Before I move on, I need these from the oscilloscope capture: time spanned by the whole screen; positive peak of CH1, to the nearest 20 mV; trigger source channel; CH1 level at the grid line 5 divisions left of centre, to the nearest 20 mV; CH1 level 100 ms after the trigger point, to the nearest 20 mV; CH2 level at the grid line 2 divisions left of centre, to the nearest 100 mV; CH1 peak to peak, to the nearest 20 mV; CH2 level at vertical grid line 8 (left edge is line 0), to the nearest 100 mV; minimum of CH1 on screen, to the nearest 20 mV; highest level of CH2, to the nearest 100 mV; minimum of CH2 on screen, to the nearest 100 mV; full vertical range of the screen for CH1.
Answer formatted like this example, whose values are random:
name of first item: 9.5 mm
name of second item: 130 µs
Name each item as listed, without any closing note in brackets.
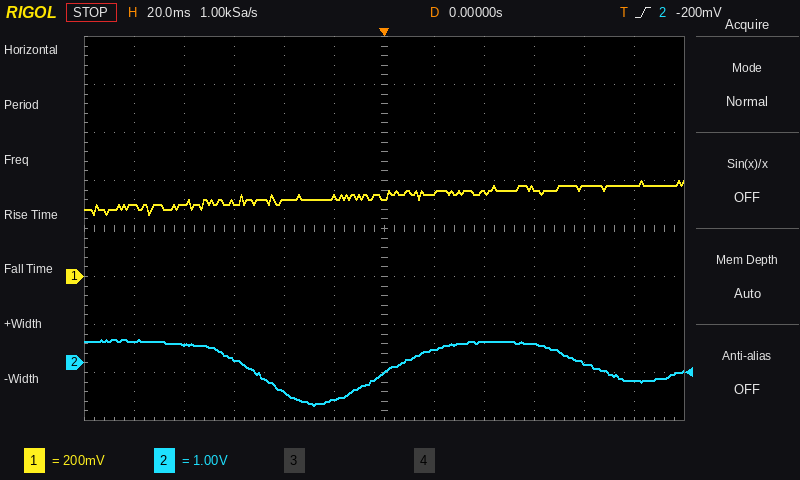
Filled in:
time spanned by the whole screen: 240 ms
positive peak of CH1, to the nearest 20 mV: 400 mV
trigger source channel: CH2
CH1 level at the grid line 5 divisions left of centre, to the nearest 20 mV: 300 mV
CH1 level 100 ms after the trigger point, to the nearest 20 mV: 380 mV
CH2 level at the grid line 2 divisions left of centre, to the nearest 100 mV: -600 mV
CH1 peak to peak, to the nearest 20 mV: 140 mV
CH2 level at vertical grid line 8 (left edge is line 0), to the nearest 100 mV: 400 mV
minimum of CH1 on screen, to the nearest 20 mV: 260 mV
highest level of CH2, to the nearest 100 mV: 500 mV
minimum of CH2 on screen, to the nearest 100 mV: -900 mV
full vertical range of the screen for CH1: 1.6 V
